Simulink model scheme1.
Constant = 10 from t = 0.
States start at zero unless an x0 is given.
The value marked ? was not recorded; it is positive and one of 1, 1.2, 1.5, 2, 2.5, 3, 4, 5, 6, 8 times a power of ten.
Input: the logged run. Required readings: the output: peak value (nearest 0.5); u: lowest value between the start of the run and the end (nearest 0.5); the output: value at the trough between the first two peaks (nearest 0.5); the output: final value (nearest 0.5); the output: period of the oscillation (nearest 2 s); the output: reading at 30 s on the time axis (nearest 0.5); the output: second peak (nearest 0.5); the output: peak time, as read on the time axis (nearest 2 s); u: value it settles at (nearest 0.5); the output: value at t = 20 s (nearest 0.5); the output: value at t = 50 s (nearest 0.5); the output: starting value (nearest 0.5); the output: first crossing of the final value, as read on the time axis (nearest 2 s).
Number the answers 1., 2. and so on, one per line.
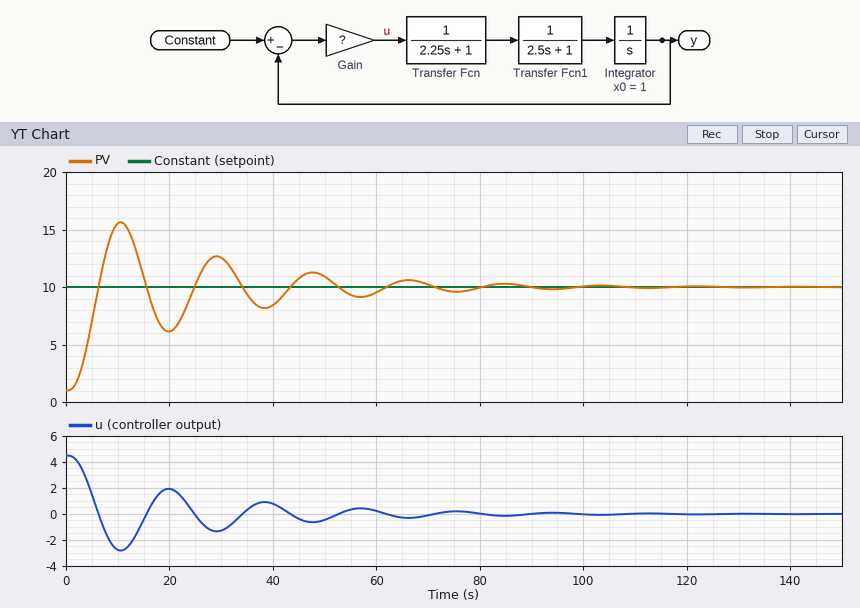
1. 15.5
2. -3.0
3. 6.0
4. 10.0
5. 18 s
6. 12.5
7. 12.5
8. 10 s
9. 0.0
10. 6.0
11. 11.0
12. 1.0
13. 6 s
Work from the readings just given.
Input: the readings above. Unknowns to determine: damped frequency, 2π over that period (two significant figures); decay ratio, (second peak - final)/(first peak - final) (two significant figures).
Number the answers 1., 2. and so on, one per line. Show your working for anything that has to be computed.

1. 2π / 18 = 0.35 rad/s
2. (12.5 - 10) / (15.5 - 10) = 0.45
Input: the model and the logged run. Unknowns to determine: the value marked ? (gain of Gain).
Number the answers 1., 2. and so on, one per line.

1. 0.5
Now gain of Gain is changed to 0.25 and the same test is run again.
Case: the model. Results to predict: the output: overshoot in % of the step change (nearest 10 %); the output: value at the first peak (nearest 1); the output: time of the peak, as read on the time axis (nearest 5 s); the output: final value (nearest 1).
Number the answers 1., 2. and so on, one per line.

1. 30 %
2. 13
3. 15 s
4. 10
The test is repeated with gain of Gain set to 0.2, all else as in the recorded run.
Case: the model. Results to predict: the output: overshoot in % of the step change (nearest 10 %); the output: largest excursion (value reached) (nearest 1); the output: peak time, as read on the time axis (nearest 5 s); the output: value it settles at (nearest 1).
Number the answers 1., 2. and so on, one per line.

1. 20 %
2. 12
3. 15 s
4. 10
